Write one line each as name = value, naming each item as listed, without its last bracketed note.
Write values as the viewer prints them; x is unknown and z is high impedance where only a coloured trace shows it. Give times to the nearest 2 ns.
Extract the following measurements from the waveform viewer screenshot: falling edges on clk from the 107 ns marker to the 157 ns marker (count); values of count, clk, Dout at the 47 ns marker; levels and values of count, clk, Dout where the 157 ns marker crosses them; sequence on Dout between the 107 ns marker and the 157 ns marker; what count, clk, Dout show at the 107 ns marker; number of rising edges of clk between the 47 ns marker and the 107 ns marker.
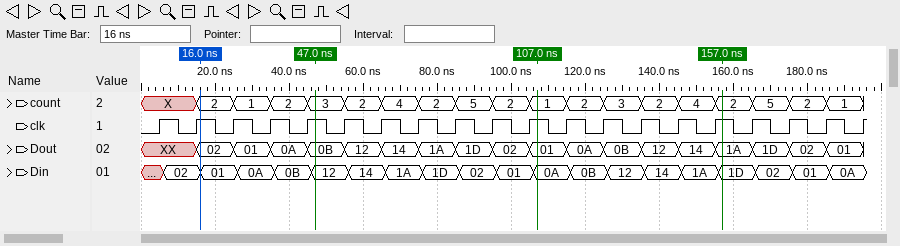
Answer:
falling edges on clk from the 107 ns marker to the 157 ns marker = 5
values of count, clk, Dout at the 47 ns marker = count=3, clk=1, Dout=0B
levels and values of count, clk, Dout where the 157 ns marker crosses them = count=2, clk=1, Dout=1A
sequence on Dout between the 107 ns marker and the 157 ns marker = 01, 0A, 0B, 12, 14, 1A
what count, clk, Dout show at the 107 ns marker = count=1, clk=1, Dout=01
number of rising edges of clk between the 47 ns marker and the 107 ns marker = 6
